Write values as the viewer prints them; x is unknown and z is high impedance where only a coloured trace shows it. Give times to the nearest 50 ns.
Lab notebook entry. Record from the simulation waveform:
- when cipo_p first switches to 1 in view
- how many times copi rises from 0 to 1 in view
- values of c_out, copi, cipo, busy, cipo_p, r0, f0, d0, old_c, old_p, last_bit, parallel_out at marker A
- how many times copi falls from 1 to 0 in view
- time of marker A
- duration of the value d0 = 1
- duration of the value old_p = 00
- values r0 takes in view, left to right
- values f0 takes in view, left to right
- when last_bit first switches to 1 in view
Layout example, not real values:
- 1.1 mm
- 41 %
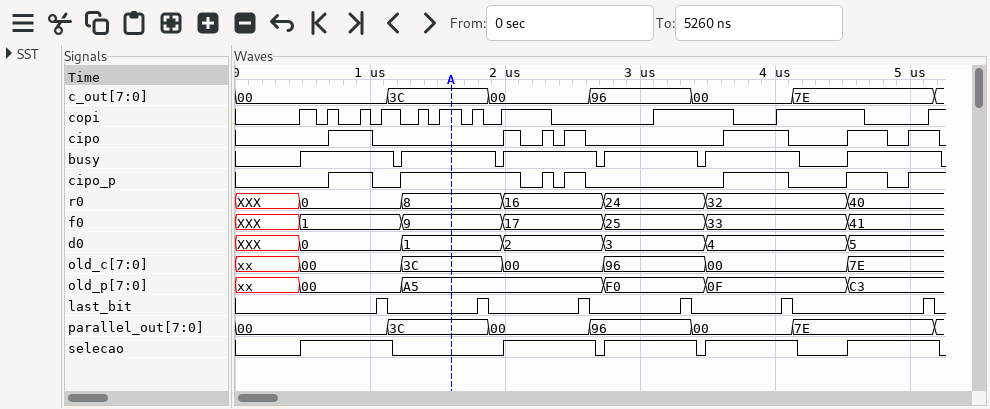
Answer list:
- 700 ns
- 11
- c_out=3C, copi=1, cipo=0, busy=1, cipo_p=1, r0=8, f0=9, d0=1, old_c=3C, old_p=A5, last_bit=0, parallel_out=3C
- 10
- 1600 ns
- 750 ns
- 750 ns
- XXX, 0, 8, 16, 24, 32, 40
- XXX, 1, 9, 17, 25, 33, 41
- 1050 ns
